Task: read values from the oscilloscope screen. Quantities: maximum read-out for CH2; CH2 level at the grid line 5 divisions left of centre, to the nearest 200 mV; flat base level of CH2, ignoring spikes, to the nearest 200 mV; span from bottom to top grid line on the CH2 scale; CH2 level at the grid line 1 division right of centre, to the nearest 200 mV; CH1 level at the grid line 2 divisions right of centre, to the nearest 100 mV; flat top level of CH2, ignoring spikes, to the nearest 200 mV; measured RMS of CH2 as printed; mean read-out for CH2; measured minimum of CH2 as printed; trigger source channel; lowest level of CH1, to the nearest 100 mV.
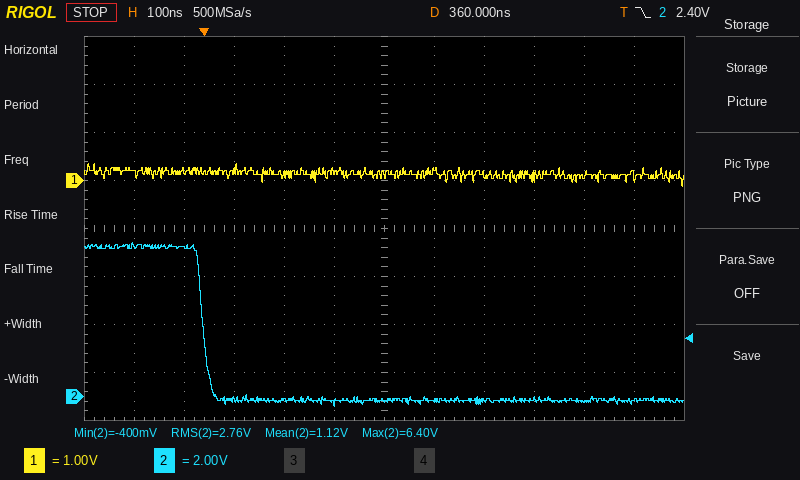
6.40 V
6.2 V
-200 mV
16 V
-200 mV
100 mV
6.2 V
2.76 V
1.12 V
-400 mV
CH2
-100 mV
